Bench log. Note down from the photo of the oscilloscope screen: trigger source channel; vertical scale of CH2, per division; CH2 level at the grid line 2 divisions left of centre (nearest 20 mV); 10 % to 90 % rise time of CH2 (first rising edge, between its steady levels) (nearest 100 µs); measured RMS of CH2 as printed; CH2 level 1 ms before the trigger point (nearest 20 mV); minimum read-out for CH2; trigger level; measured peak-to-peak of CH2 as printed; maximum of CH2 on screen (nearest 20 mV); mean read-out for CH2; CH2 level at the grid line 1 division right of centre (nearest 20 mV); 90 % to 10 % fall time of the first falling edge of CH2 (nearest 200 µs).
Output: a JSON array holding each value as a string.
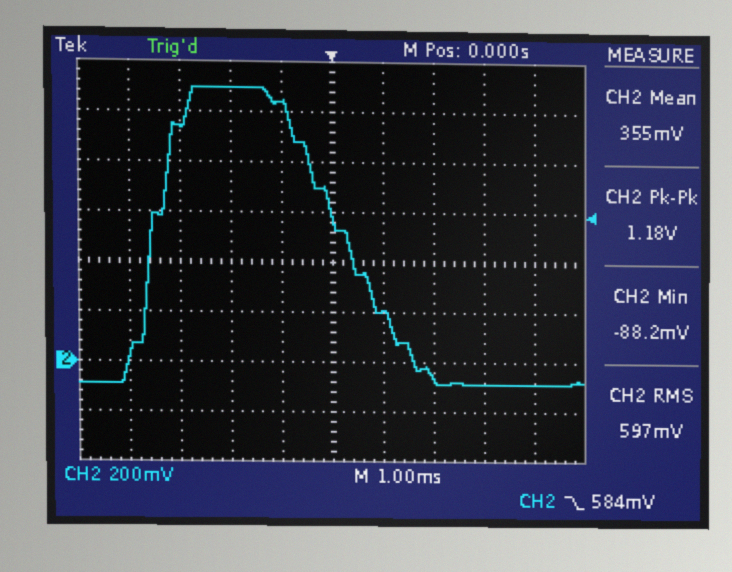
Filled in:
["CH2", "200 mV", "1.10 V", "1.1 ms", "597 mV", "1.04 V", "-88.2 mV", "584 mV", "1.18 V", "1.10 V", "355 mV", "200 mV", "2.4 ms"]
